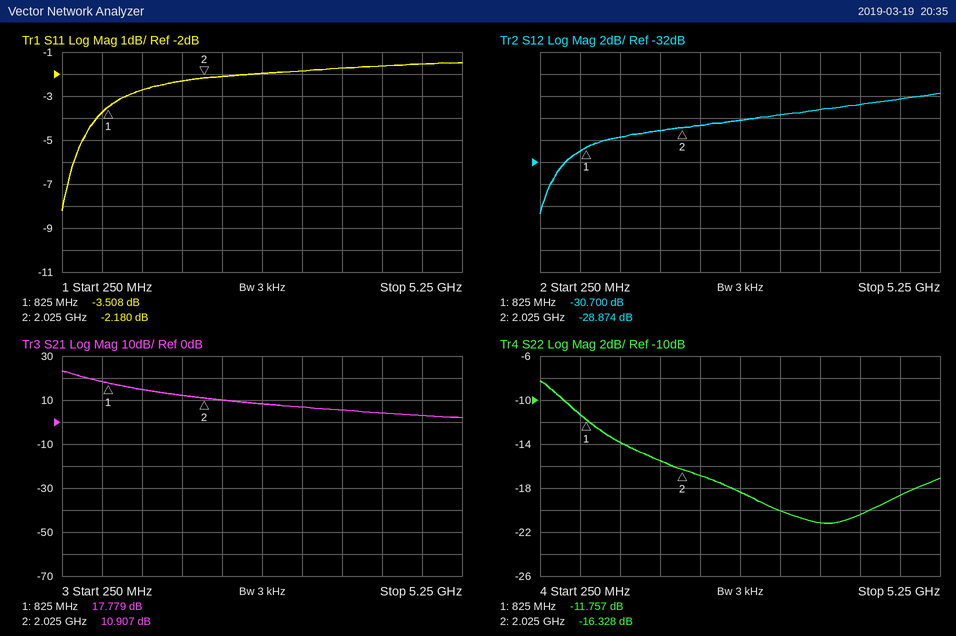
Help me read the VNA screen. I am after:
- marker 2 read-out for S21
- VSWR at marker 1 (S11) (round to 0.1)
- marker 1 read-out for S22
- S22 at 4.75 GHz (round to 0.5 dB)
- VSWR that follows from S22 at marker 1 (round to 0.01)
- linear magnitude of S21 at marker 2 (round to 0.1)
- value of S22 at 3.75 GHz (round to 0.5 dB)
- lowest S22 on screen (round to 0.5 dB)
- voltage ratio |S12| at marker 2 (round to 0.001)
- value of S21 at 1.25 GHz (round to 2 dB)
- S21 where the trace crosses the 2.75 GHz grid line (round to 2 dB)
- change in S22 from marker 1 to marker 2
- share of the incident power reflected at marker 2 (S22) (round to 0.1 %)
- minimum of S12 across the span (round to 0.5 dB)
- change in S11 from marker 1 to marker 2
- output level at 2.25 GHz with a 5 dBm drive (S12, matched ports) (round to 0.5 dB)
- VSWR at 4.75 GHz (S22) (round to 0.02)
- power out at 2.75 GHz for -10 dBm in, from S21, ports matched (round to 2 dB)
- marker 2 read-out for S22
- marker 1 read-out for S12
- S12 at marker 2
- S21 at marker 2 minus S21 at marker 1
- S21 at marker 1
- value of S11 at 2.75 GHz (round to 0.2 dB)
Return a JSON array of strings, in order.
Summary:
["10.907 dB", "5.0", "-11.757 dB", "-18.5 dB", "1.70", "3.5", "-21.0 dB", "-21.0 dB", "0.036", "14 dB", "8 dB", "-4.571 dB", "2.3 %", "-36.5 dB", "1.328 dB", "-23.5 dBm", "1.26", "-2 dBm", "-16.328 dB", "-30.700 dB", "-28.874 dB", "-6.872 dB", "17.779 dB", "-2.0 dB"]
